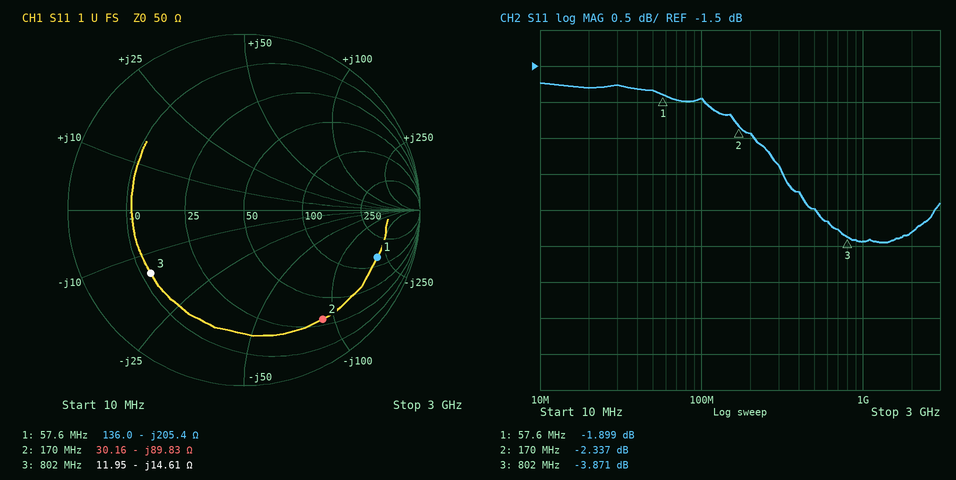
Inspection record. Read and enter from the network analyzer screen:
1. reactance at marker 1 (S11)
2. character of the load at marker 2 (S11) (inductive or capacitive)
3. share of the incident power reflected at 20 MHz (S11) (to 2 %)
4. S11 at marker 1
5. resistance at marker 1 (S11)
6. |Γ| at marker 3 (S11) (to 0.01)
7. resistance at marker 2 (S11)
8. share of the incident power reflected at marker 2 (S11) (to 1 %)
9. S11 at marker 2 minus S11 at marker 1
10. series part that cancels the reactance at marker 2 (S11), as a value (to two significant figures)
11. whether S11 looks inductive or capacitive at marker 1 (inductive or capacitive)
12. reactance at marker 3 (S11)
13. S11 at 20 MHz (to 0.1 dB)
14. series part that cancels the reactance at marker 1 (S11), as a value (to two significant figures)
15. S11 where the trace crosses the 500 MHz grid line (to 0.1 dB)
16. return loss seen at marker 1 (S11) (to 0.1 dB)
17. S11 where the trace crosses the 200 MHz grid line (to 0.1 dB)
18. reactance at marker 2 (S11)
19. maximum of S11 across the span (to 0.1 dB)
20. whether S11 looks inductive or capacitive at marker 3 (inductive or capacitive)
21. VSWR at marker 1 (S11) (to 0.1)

-205.4 Ω
capacitive
66 %
-1.899 dB
136.0 Ω
0.64
30.16 Ω
58 %
-0.438 dB
84 nH
capacitive
-14.61 Ω
-1.8 dB
570 nH
-3.5 dB
1.9 dB
-2.4 dB
-89.83 Ω
-1.7 dB
capacitive
9.2
